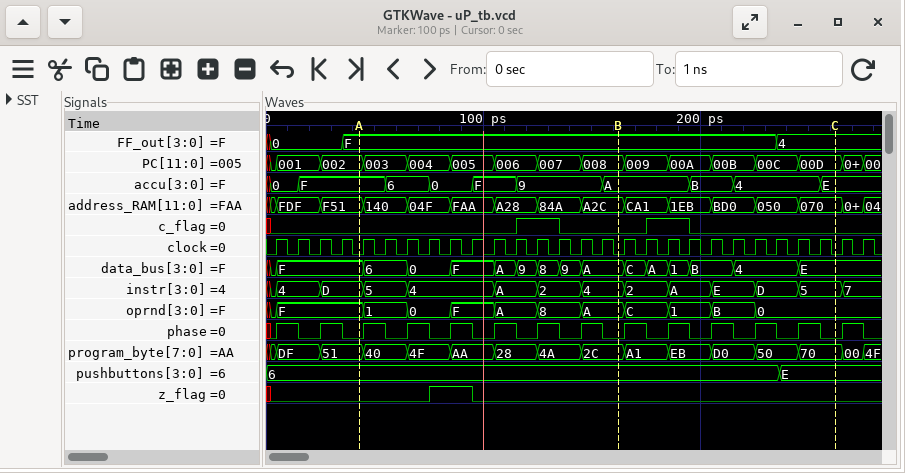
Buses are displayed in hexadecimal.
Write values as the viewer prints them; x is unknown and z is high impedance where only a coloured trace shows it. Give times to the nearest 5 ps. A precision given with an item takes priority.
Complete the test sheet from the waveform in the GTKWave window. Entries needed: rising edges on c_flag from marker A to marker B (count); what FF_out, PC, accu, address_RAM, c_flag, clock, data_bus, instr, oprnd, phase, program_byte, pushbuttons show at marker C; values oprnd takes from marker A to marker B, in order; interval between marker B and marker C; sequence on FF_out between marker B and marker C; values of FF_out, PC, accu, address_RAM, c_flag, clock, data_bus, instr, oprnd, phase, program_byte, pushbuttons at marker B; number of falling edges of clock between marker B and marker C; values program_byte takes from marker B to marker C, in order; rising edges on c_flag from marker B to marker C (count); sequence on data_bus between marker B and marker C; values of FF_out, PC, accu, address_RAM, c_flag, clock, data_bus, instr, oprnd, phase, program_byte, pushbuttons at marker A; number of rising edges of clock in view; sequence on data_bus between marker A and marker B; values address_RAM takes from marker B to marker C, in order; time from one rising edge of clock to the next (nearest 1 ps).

1
FF_out=4, PC=00D, accu=E, address_RAM=070, c_flag=0, clock=0, data_bus=E, instr=5, oprnd=0, phase=0, program_byte=70, pushbuttons=E
F, 1, 0, F, A, 8, A
100 ps
F, 4
FF_out=F, PC=008, accu=A, address_RAM=A2C, c_flag=0, clock=0, data_bus=A, instr=4, oprnd=A, phase=0, program_byte=2C, pushbuttons=6
10
2C, A1, EB, D0, 50, 70
1
A, C, A, 1, B, 4, E
FF_out=F, PC=002, accu=F, address_RAM=F51, c_flag=0, clock=0, data_bus=F, instr=D, oprnd=F, phase=0, program_byte=51, pushbuttons=6
28
F, 6, 0, F, A, 9, 8, 9, A
A2C, CA1, 1EB, BD0, 050, 070
10 ps
